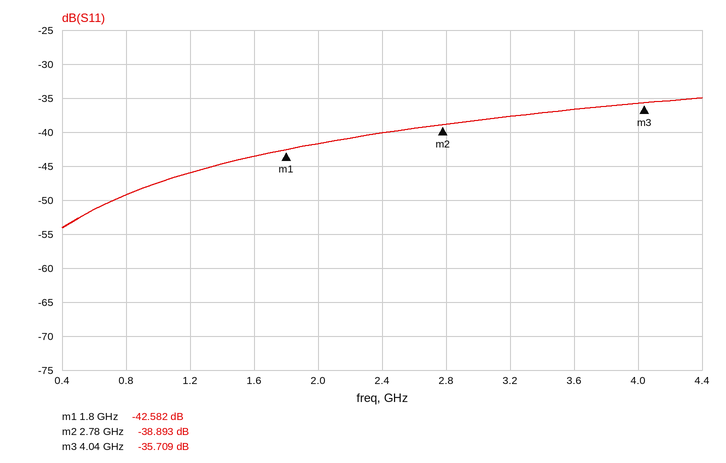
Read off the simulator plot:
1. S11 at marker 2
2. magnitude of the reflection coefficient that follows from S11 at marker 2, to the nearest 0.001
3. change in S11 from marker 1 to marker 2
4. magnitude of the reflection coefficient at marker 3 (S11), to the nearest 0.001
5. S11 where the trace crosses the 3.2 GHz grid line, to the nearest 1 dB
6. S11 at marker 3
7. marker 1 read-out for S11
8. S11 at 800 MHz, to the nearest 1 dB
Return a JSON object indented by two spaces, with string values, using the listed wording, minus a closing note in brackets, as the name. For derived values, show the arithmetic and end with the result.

{
  "S11 at marker 2": "-38.893 dB",
  "magnitude of the reflection coefficient that follows from S11 at marker 2, to the nearest 0.001": "10^(-38.893/20) ≈ 0.011",
  "change in S11 from marker 1 to marker 2": "-38.893 − (-42.582) = 3.689 dB",
  "magnitude of the reflection coefficient at marker 3 (S11), to the nearest 0.001": "10^(-35.709/20) ≈ 0.016",
  "S11 where the trace crosses the 3.2 GHz grid line, to the nearest 1 dB": "-38 dB",
  "S11 at marker 3": "-35.709 dB",
  "marker 1 read-out for S11": "-42.582 dB",
  "S11 at 800 MHz, to the nearest 1 dB": "-49 dB"
}
